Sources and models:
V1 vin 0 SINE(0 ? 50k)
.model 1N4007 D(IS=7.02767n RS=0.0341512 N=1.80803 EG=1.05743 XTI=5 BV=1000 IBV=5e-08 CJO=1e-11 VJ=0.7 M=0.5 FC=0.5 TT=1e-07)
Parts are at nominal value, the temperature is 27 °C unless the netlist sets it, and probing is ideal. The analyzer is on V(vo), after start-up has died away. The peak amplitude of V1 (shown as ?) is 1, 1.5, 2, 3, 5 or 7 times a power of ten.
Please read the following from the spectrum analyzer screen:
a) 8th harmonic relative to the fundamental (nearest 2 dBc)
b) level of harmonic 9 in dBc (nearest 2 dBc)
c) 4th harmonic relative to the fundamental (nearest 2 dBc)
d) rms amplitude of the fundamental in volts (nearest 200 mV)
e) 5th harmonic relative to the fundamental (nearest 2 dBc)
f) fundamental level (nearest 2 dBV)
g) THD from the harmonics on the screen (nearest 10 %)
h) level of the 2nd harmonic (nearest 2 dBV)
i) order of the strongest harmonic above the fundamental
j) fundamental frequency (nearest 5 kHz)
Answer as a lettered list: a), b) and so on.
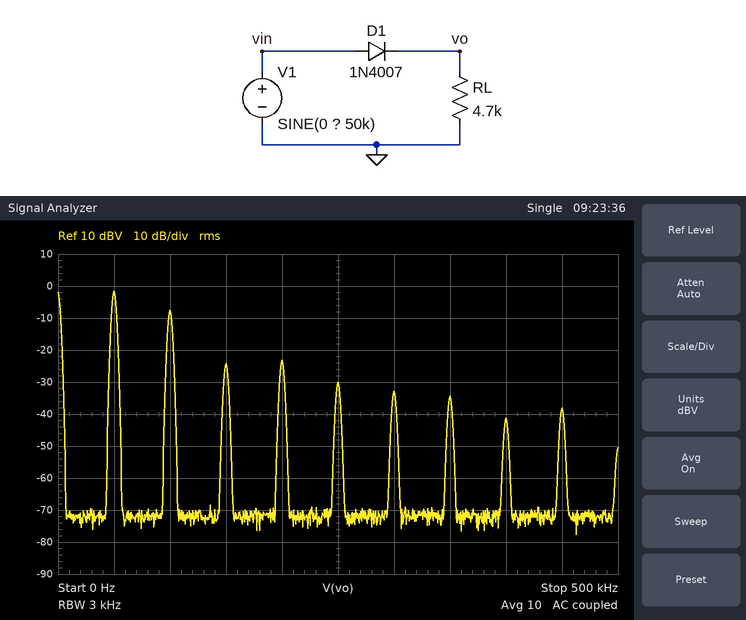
a) -40 dBc
b) -36 dBc
c) -22 dBc
d) 800 mV
e) -28 dBc
f) -2 dBV
g) 50 %
h) -8 dBV
i) 2
j) 50 kHz
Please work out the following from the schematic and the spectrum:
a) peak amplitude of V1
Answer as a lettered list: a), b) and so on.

a) 3 V
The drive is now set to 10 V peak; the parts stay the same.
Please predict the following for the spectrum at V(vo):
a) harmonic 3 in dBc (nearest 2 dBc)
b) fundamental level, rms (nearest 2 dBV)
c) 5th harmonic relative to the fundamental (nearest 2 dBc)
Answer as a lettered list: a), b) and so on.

a) -32 dBc
b) 10 dBV
c) -38 dBc
